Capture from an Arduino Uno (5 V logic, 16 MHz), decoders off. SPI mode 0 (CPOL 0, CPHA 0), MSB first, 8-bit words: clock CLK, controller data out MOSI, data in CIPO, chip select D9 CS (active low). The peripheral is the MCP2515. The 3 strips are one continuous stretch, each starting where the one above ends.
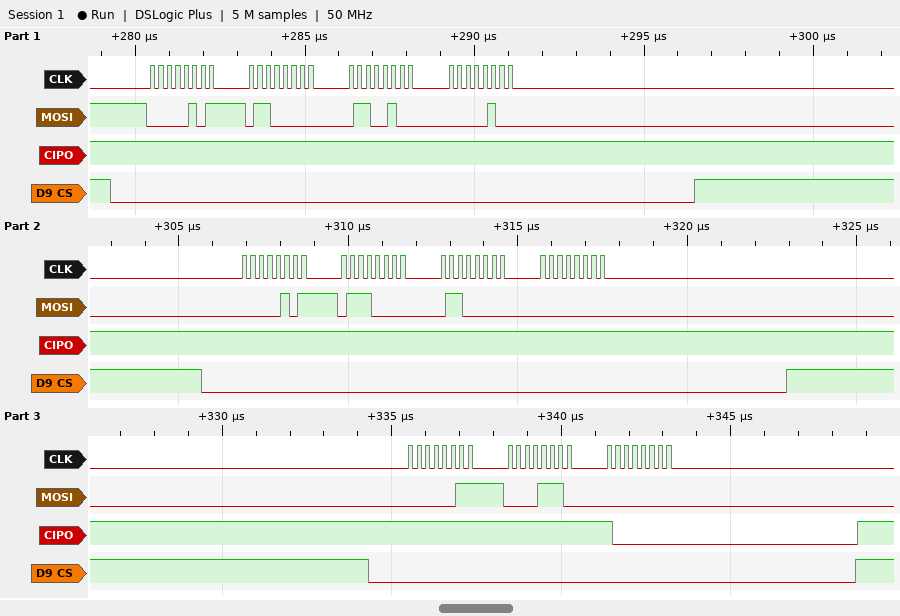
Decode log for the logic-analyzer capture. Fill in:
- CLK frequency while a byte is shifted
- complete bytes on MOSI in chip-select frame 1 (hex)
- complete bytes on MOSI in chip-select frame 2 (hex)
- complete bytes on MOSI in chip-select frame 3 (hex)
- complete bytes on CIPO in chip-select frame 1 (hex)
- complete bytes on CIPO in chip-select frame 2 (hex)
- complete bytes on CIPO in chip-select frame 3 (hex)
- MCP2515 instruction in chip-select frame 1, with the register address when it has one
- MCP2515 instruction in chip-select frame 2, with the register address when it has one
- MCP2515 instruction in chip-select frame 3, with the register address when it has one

4 MHz
0x05 0x60 0x64 0x04
0x05 0x70 0x60 0x00
0x03 0x0E 0x00
0xFF 0xFF 0xFF 0xFF
0xFF 0xFF 0xFF 0xFF
0xFF 0xFF 0x80
BIT MODIFY 0x60
BIT MODIFY 0x70
READ 0x0E
